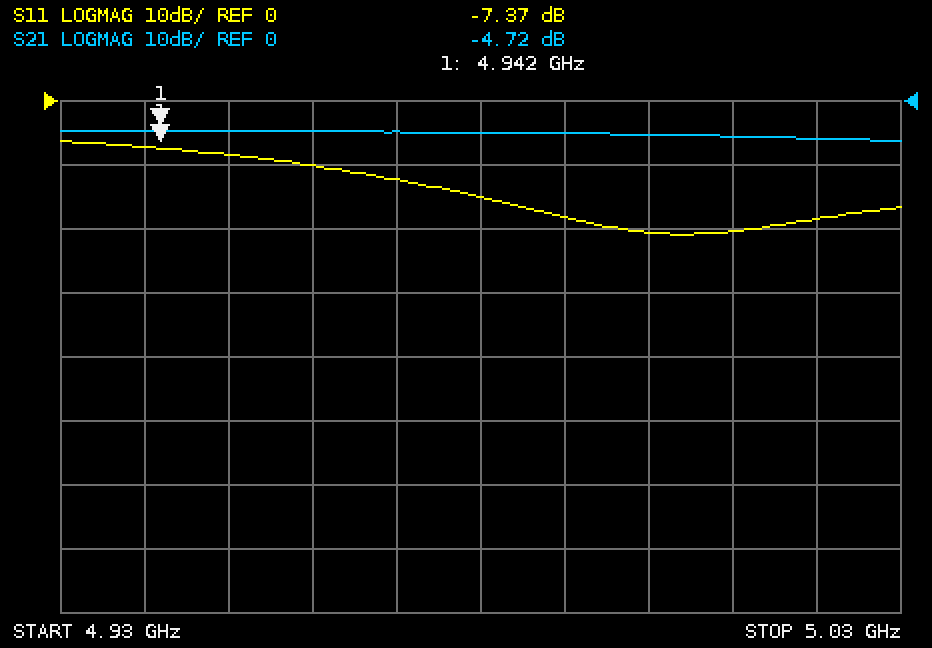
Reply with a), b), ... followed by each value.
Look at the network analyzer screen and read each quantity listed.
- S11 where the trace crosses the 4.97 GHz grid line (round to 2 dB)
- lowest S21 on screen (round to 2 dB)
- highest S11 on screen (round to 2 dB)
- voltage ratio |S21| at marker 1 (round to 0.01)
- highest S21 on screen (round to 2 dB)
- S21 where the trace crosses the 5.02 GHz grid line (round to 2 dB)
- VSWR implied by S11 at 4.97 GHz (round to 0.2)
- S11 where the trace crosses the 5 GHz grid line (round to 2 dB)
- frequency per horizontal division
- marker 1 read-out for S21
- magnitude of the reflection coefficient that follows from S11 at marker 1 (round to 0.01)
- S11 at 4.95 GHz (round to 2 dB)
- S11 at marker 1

a) -12 dB
b) -6 dB
c) -6 dB
d) 0.58
e) -4 dB
f) -6 dB
g) 1.6
h) -20 dB
i) 10 MHz
j) -4.72 dB
k) 0.43
l) -8 dB
m) -7.37 dB
